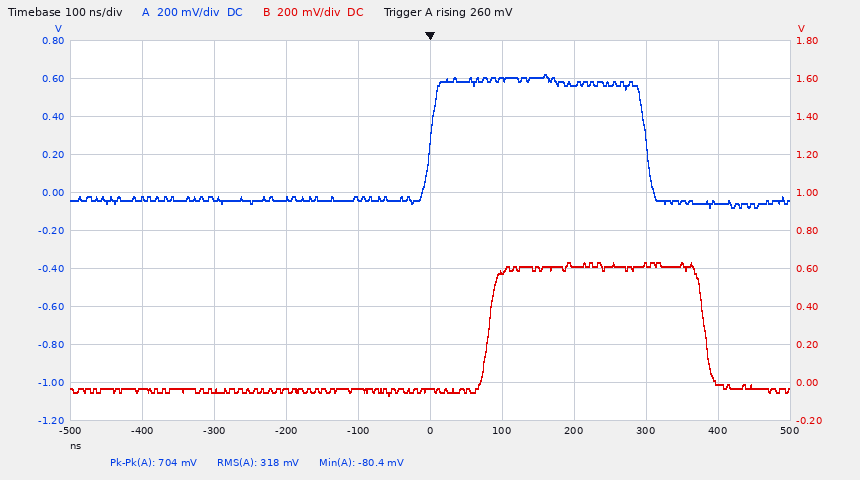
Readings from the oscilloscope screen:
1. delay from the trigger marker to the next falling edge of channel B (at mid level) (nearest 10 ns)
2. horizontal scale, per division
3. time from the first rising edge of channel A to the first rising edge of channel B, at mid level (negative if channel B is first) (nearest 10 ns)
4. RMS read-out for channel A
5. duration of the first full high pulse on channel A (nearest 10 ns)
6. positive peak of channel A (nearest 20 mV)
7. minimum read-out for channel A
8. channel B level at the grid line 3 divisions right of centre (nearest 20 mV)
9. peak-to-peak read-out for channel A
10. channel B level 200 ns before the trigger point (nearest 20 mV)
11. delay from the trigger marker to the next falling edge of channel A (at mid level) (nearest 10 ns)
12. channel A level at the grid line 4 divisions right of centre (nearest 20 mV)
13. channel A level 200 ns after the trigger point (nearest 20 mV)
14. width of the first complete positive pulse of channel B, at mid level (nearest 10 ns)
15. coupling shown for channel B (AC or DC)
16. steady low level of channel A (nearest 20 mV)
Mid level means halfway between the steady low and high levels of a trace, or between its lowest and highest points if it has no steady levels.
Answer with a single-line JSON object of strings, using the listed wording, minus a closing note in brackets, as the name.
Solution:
{"delay from the trigger marker to the next falling edge of channel B (at mid level)": "380 ns", "horizontal scale, per division": "100 ns", "time from the first rising edge of channel A to the first rising edge of channel B, at mid level (negative if channel B is first)": "+80 ns", "RMS read-out for channel A": "318 mV", "duration of the first full high pulse on channel A": "300 ns", "positive peak of channel A": "620 mV", "minimum read-out for channel A": "-80.4 mV", "channel B level at the grid line 3 divisions right of centre": "620 mV", "peak-to-peak read-out for channel A": "704 mV", "channel B level 200 ns before the trigger point": "-40 mV", "delay from the trigger marker to the next falling edge of channel A (at mid level)": "300 ns", "channel A level at the grid line 4 divisions right of centre": "-60 mV", "channel A level 200 ns after the trigger point": "560 mV", "width of the first complete positive pulse of channel B, at mid level": "300 ns", "coupling shown for channel B": "DC", "steady low level of channel A": "-40 mV"}
